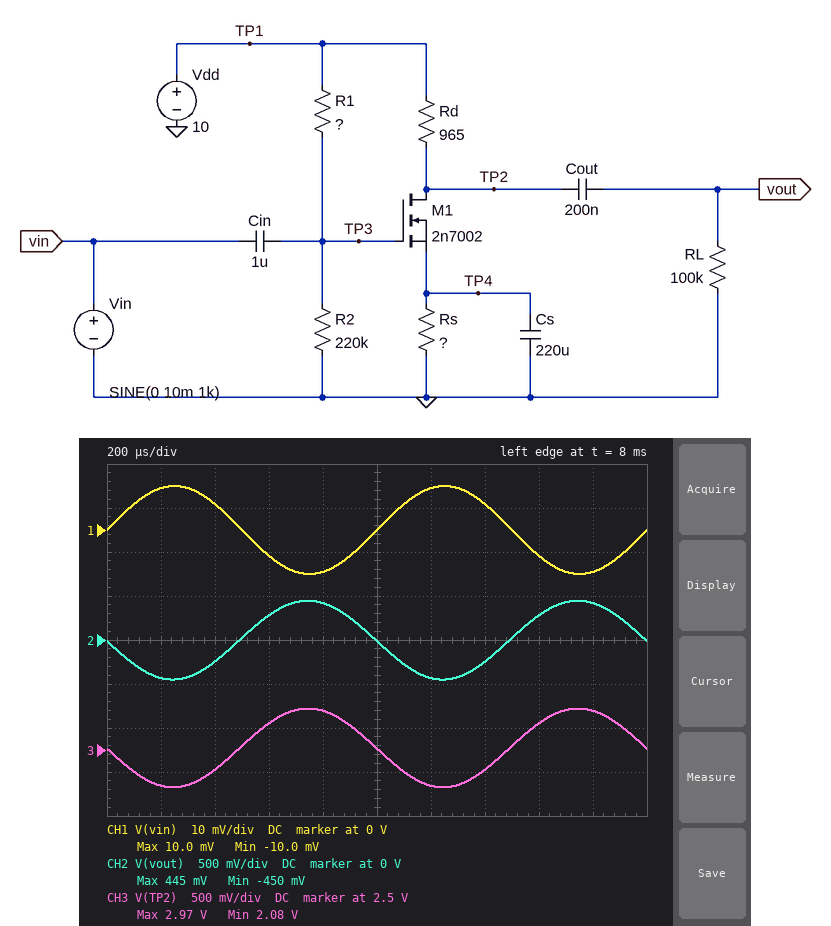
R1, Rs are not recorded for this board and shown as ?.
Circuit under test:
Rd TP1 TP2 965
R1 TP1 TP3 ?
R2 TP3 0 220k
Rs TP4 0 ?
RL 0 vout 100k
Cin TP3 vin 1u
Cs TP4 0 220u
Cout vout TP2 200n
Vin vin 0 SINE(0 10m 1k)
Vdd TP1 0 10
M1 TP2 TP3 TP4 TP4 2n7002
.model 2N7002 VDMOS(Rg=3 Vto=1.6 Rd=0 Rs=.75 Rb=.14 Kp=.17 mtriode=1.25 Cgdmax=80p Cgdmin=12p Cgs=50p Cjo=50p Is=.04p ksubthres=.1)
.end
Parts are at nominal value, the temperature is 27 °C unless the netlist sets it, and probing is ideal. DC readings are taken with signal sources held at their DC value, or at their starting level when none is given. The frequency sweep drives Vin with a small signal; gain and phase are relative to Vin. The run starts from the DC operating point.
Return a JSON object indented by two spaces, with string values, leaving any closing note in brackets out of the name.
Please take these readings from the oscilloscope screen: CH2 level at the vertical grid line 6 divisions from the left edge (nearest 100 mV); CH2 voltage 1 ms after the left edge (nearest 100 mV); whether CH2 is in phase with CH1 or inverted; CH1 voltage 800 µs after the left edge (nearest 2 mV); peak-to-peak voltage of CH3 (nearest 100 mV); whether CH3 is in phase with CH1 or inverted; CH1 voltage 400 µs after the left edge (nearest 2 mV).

{
  "CH2 level at the vertical grid line 6 divisions from the left edge": "-400 mV",
  "CH2 voltage 1 ms after the left edge": "0 V",
  "whether CH2 is in phase with CH1 or inverted": "inverted",
  "CH1 voltage 800 µs after the left edge": "-10 mV",
  "peak-to-peak voltage of CH3": "900 mV",
  "whether CH3 is in phase with CH1 or inverted": "inverted",
  "CH1 voltage 400 µs after the left edge": "6 mV"
}
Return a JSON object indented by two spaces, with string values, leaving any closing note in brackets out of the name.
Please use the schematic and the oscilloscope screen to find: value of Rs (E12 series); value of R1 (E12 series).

{
  "value of Rs": "220 Ω",
  "value of R1": "390 kΩ"
}
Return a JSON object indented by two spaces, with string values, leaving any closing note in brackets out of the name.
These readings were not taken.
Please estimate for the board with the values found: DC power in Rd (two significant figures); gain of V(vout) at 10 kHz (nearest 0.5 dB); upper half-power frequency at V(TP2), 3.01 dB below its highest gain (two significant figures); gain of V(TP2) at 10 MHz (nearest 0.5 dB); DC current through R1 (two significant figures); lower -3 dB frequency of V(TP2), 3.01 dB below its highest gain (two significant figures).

{
  "DC power in Rd": "58 mW",
  "gain of V(vout) at 10 kHz": "33.0 dB",
  "upper half-power frequency at V(TP2), 3.01 dB below its highest gain": "1.4 MHz",
  "gain of V(TP2) at 10 MHz": "16.0 dB",
  "DC current through R1": "16 µA",
  "lower -3 dB frequency of V(TP2), 3.01 dB below its highest gain": "37 Hz"
}
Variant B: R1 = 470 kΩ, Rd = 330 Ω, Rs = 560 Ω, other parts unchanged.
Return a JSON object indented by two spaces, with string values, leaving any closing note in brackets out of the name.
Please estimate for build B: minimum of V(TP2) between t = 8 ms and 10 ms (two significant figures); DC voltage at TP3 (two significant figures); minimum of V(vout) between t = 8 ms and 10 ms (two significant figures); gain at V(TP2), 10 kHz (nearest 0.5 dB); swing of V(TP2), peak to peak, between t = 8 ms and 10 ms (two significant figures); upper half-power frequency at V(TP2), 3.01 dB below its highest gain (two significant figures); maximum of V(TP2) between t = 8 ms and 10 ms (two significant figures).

{
  "minimum of V(TP2) between t = 8 ms and 10 ms": "9.1 V",
  "DC voltage at TP3": "3.2 V",
  "minimum of V(vout) between t = 8 ms and 10 ms": "-79 mV",
  "gain at V(TP2), 10 kHz": "18.0 dB",
  "swing of V(TP2), peak to peak, between t = 8 ms and 10 ms": "160 mV",
  "upper half-power frequency at V(TP2), 3.01 dB below its highest gain": "15 MHz",
  "maximum of V(TP2) between t = 8 ms and 10 ms": "9.2 V"
}
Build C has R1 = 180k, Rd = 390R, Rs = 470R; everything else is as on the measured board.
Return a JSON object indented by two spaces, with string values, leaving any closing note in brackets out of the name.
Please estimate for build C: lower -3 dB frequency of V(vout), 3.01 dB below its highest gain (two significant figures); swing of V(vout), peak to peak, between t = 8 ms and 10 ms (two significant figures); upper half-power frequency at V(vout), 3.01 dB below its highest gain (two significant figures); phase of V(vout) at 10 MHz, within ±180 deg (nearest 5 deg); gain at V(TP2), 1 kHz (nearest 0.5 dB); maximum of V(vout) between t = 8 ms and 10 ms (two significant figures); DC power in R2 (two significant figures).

{
  "lower -3 dB frequency of V(vout), 3.01 dB below its highest gain": "37 Hz",
  "swing of V(vout), peak to peak, between t = 8 ms and 10 ms": "360 mV",
  "upper half-power frequency at V(vout), 3.01 dB below its highest gain": "7.7 MHz",
  "phase of V(vout) at 10 MHz, within ±180 deg": "125 deg",
  "gain at V(TP2), 1 kHz": "25.0 dB",
  "maximum of V(vout) between t = 8 ms and 10 ms": "180 mV",
  "DC power in R2": "140 µW"
}
